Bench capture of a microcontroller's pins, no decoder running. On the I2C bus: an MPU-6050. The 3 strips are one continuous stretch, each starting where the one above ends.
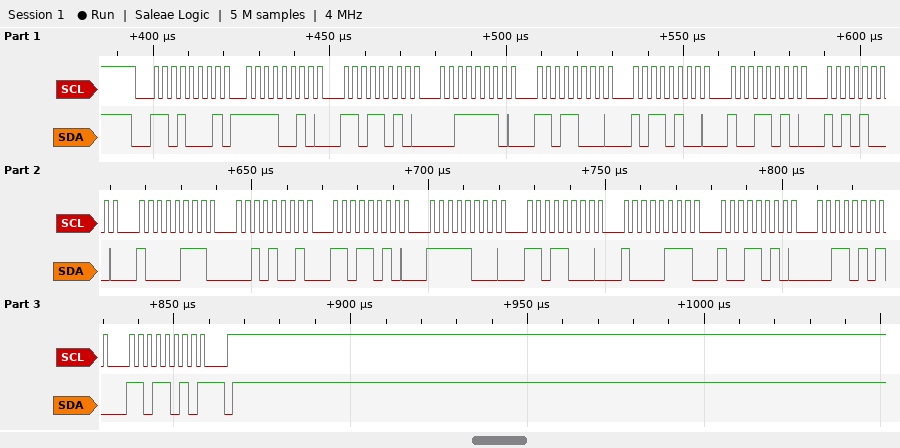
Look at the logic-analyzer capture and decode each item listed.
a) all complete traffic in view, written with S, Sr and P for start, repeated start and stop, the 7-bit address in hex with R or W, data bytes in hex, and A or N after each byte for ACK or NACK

S 68R A F2 A DA A 3E A D8 A B4 A 9A A A8 A 87 A 29 A DA A F8 A D8 A 87 A 9A A 35 A DA N P
